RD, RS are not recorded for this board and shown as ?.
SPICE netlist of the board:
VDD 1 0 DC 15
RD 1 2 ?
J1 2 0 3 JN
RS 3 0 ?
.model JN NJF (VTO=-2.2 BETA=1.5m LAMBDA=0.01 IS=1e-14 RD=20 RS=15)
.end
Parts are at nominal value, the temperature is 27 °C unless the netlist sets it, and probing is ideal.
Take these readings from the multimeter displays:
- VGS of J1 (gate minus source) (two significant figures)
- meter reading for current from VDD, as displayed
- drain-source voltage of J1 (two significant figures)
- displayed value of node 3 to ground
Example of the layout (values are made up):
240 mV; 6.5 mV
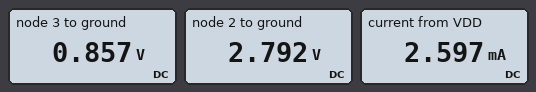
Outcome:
-860 mV; 2.597 mA; 1.9 V; 0.857 V
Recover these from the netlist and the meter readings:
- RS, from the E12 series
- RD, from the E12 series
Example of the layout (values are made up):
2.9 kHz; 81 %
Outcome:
330 Ω; 4.7 kΩ
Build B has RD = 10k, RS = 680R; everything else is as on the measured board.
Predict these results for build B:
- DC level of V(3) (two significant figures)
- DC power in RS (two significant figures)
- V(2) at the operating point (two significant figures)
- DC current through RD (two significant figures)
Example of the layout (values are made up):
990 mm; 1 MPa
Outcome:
920 mV; 1.3 mW; 1.4 V; 1.4 mA
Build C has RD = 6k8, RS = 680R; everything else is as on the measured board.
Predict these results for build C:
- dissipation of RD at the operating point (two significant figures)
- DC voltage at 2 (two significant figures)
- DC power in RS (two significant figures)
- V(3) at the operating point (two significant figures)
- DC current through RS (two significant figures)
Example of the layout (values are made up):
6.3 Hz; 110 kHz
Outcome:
19 mW; 3.7 V; 1.9 mW; 1.1 V; 1.7 mA
